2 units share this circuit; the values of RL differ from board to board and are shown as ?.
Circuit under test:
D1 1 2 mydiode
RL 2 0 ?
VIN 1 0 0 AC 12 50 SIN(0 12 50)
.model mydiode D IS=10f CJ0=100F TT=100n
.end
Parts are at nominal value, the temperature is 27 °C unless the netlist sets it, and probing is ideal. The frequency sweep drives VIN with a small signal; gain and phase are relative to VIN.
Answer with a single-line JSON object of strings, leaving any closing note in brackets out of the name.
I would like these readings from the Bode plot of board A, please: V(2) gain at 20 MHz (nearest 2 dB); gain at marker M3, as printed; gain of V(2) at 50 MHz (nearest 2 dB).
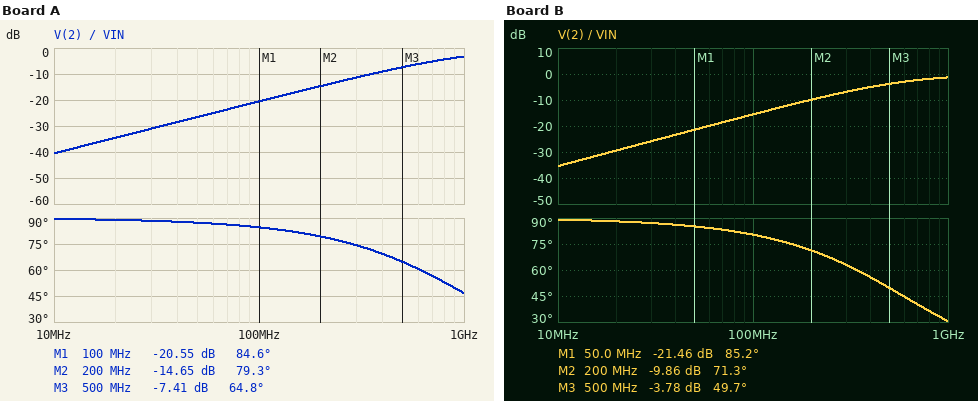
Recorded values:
{"V(2) gain at 20 MHz": "-34 dB", "gain at marker M3, as printed": "-7.41 dB", "gain of V(2) at 50 MHz": "-26 dB"}
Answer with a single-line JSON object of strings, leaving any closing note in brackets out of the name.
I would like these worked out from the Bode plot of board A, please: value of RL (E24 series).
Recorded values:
{"value of RL": "1.5 kΩ"}
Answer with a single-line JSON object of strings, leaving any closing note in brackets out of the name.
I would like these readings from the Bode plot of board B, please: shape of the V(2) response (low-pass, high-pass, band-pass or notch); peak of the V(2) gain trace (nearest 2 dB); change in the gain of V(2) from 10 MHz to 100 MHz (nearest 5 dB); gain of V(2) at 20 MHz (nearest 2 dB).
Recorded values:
{"shape of the V(2) response": "high-pass", "peak of the V(2) gain trace": "-2 dB", "change in the gain of V(2) from 10 MHz to 100 MHz": "20 dB", "gain of V(2) at 20 MHz": "-30 dB"}
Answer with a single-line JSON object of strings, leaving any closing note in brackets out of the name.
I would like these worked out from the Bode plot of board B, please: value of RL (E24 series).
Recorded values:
{"value of RL": "2.7 kΩ"}
